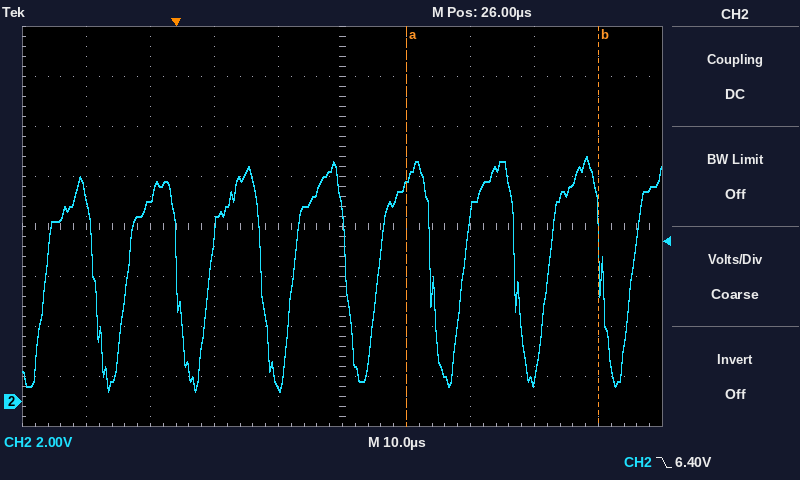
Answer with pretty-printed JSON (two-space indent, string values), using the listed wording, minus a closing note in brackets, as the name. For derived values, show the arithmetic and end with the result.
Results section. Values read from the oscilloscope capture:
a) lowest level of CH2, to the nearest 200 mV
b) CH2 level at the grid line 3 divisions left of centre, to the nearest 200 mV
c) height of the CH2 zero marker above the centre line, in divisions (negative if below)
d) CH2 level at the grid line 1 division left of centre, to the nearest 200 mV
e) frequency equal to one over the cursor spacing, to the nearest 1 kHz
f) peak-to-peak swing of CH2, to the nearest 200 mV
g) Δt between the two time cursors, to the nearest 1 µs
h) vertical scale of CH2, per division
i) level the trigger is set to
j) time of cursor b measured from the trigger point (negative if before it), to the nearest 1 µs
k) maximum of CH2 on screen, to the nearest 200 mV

{
  "lowest level of CH2, to the nearest 200 mV": "400 mV",
  "CH2 level at the grid line 3 divisions left of centre, to the nearest 200 mV": "8.2 V",
  "height of the CH2 zero marker above the centre line, in divisions": "-3.5 div",
  "CH2 level at the grid line 1 division left of centre, to the nearest 200 mV": "600 mV",
  "frequency equal to one over the cursor spacing, to the nearest 1 kHz": "1 / 30 µs ≈ 33 kHz",
  "peak-to-peak swing of CH2, to the nearest 200 mV": "9.8 V − (400 mV) = 9.4 V",
  "Δt between the two time cursors, to the nearest 1 µs": "30 µs",
  "vertical scale of CH2, per division": "2 V",
  "level the trigger is set to": "6.40 V",
  "time of cursor b measured from the trigger point (negative if before it), to the nearest 1 µs": "+66 µs",
  "maximum of CH2 on screen, to the nearest 200 mV": "9.8 V"
}
